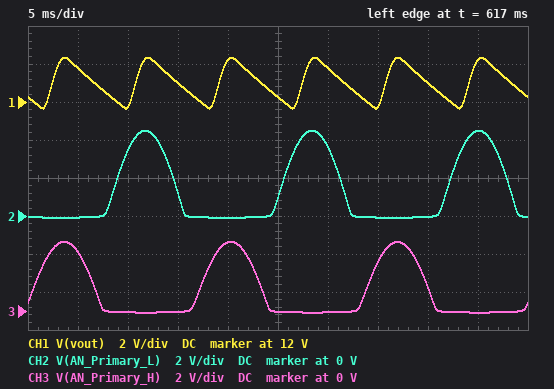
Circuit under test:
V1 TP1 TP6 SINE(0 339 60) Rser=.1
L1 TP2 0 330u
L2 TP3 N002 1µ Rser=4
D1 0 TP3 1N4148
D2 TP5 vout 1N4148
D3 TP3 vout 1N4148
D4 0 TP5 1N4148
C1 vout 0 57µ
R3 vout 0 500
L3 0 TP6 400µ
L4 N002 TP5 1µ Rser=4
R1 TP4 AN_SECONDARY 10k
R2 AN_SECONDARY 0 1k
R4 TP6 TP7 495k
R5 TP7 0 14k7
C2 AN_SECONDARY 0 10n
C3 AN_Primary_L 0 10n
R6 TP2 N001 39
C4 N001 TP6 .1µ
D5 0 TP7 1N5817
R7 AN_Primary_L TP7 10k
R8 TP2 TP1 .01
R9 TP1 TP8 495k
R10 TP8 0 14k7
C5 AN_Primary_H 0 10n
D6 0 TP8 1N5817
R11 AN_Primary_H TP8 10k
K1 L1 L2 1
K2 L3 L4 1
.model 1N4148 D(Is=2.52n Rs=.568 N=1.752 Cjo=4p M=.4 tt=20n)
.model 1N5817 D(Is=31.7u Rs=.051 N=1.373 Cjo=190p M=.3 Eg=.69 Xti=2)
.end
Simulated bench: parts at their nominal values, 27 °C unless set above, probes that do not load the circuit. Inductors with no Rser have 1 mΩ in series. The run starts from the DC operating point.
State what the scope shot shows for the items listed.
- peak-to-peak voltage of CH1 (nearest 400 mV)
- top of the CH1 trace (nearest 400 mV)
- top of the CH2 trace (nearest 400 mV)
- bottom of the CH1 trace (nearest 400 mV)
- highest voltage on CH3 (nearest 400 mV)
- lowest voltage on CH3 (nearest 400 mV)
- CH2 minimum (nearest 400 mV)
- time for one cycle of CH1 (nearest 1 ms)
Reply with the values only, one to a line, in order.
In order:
2.8 V
14.4 V
4.4 V
11.6 V
3.6 V
0 V
0 V
8 ms
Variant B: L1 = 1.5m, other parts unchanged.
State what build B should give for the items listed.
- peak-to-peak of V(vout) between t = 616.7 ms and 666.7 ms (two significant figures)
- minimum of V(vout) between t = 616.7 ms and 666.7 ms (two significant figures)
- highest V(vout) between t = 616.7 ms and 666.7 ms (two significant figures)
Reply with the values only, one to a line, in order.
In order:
1.6 V
6.9 V
8.5 V
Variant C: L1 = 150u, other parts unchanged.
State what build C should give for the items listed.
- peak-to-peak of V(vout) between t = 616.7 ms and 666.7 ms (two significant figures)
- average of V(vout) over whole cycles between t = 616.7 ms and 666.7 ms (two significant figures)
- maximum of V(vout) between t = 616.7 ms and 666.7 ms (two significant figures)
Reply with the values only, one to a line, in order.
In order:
2.9 V
14 V
15 V
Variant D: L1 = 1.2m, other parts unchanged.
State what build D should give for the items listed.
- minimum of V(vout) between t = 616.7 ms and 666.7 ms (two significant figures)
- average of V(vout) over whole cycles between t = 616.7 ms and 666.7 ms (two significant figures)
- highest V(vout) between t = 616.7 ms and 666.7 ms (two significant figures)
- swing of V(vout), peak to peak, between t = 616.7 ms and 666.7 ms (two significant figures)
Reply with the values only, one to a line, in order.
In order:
7.7 V
8.6 V
9.5 V
1.8 V
